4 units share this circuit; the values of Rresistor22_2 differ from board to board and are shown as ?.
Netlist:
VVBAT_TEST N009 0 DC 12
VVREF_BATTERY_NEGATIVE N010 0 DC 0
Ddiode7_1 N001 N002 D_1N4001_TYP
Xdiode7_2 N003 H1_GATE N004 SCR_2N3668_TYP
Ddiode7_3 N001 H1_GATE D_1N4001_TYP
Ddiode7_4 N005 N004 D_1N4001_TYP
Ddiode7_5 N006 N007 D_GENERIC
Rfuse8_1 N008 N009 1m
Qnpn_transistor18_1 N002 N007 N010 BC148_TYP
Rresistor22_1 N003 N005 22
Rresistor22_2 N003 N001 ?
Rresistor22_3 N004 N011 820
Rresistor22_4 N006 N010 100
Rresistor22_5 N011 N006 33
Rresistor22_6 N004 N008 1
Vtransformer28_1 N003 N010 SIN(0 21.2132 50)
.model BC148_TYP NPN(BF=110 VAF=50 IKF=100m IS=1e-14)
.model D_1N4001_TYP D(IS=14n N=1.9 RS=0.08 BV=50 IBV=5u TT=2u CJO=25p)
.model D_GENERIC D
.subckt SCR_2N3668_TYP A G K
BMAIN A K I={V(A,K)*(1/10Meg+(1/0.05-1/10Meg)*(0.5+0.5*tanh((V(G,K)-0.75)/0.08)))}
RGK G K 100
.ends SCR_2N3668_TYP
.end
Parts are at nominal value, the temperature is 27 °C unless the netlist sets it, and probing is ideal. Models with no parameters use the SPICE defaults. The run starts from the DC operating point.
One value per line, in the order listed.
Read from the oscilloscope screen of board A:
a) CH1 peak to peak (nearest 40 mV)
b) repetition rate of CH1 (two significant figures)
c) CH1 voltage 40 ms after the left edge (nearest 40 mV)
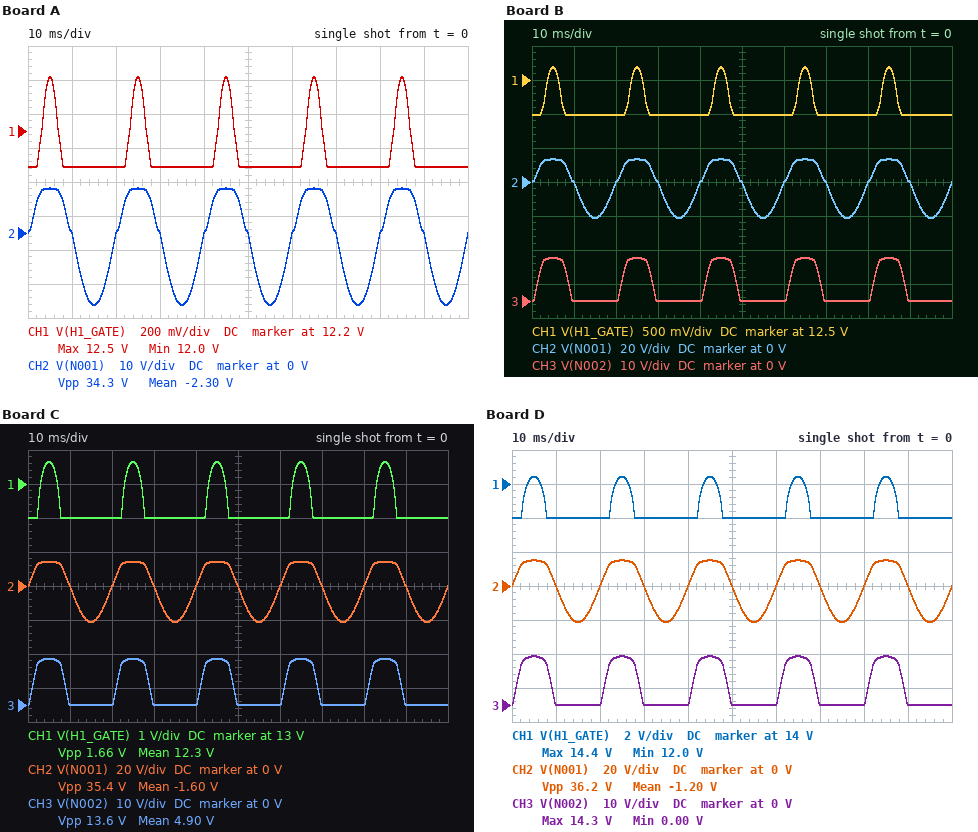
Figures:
520 mV
50 Hz
12.00 V
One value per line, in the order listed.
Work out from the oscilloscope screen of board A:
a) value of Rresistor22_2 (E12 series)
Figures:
820 Ω
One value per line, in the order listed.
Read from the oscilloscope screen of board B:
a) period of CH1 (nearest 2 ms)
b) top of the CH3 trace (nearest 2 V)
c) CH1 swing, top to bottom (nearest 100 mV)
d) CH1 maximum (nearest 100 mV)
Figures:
20 ms
12 V
700 mV
12.7 V
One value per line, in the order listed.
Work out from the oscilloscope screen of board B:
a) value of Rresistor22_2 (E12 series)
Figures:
680 Ω
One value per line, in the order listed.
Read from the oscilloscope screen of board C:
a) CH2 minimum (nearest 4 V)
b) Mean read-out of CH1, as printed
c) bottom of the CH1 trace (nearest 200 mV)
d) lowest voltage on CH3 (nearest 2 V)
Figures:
-20 V
12.3 V
12.0 V
0 V
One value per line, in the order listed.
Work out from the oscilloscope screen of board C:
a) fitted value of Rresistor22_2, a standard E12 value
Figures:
220 Ω
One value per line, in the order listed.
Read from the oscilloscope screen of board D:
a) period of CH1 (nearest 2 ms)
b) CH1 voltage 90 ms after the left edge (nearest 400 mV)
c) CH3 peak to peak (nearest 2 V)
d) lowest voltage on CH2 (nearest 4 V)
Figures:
20 ms
12.0 V
14 V
-20 V
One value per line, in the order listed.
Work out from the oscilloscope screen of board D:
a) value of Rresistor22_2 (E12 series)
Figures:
100 Ω
